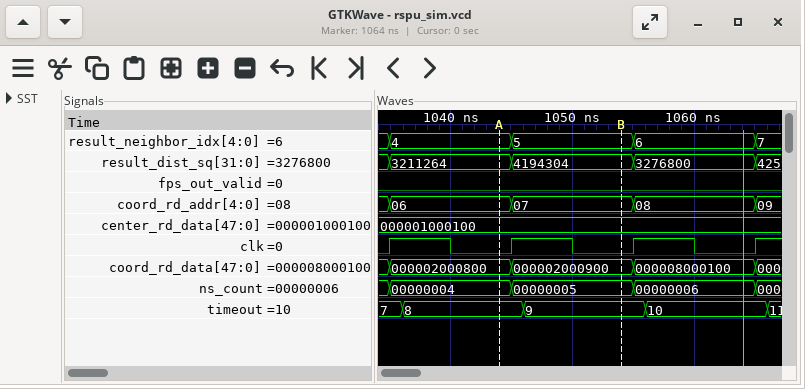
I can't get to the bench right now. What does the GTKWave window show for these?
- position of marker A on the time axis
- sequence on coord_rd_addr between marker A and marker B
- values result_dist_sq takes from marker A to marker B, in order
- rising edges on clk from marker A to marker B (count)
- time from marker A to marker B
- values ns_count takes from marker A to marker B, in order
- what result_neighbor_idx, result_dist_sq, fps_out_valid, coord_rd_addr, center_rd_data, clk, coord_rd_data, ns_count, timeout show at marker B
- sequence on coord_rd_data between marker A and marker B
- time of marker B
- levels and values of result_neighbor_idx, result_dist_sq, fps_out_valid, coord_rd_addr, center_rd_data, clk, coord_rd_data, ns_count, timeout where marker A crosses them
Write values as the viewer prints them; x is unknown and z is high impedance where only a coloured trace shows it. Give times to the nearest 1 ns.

1044 ns
06, 07
3211264, 4194304
1
10 ns
00000004, 00000005
result_neighbor_idx=5, result_dist_sq=4194304, fps_out_valid=0, coord_rd_addr=07, center_rd_data=000001000100, clk=0, coord_rd_data=000002000900, ns_count=00000005, timeout=9
000002000800, 000002000900
1054 ns
result_neighbor_idx=4, result_dist_sq=3211264, fps_out_valid=0, coord_rd_addr=06, center_rd_data=000001000100, clk=0, coord_rd_data=000002000800, ns_count=00000004, timeout=8
